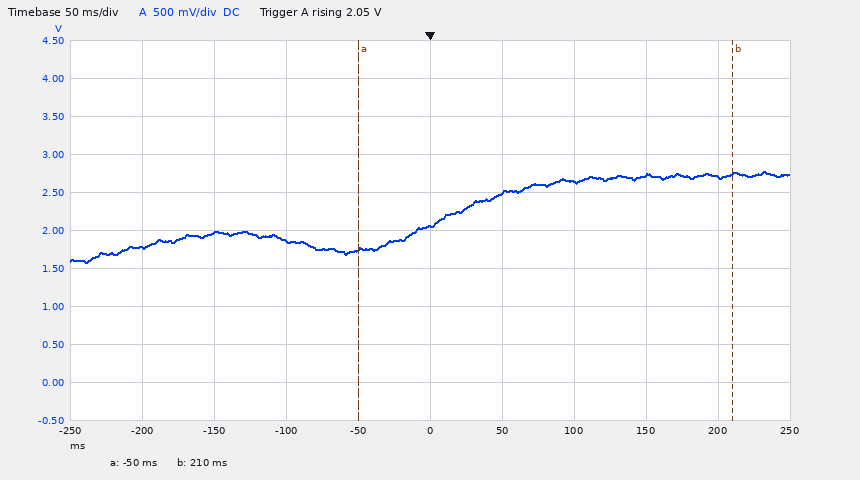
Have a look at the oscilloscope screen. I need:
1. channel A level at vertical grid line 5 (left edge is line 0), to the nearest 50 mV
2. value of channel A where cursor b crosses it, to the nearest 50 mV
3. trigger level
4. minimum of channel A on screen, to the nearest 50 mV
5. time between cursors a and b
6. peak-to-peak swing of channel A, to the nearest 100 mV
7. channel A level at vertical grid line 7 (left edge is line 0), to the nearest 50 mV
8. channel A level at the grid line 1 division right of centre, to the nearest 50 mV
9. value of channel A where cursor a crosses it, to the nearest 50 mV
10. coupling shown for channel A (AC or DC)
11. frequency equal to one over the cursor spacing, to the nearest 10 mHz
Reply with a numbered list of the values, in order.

1. 2.05 V
2. 2.75 V
3. 2.05 V
4. 1.60 V
5. 260 ms
6. 1.20 V
7. 2.65 V
8. 2.50 V
9. 1.75 V
10. DC
11. 3.85 Hz
